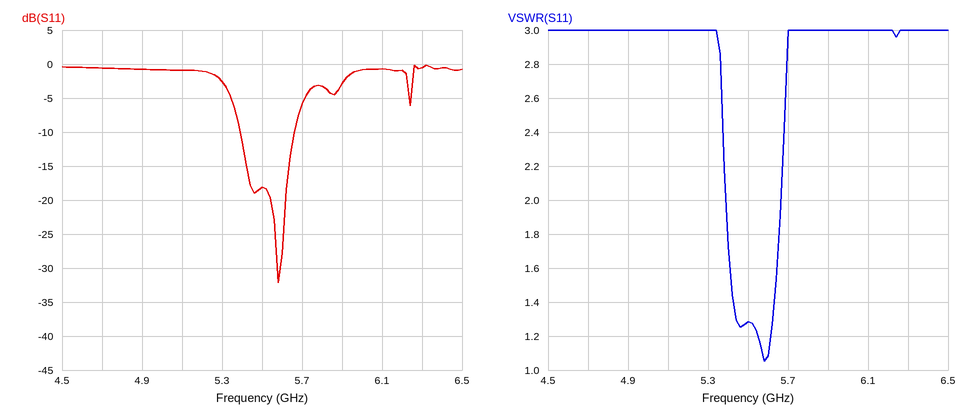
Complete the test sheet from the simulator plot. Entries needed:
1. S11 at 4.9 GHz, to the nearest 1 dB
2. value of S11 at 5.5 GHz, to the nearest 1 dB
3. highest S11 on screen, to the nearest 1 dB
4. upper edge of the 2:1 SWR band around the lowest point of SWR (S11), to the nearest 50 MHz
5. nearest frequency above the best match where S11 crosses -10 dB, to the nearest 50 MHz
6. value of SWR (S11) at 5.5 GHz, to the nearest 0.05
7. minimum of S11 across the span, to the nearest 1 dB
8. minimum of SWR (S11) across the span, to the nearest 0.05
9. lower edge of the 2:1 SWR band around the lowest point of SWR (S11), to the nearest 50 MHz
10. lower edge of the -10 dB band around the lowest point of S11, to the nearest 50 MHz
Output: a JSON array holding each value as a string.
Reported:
["-1 dB", "-18 dB", "0 dB", "5.65 GHz", "5.65 GHz", "1.30", "-32 dB", "1.05", "5.40 GHz", "5.40 GHz"]
